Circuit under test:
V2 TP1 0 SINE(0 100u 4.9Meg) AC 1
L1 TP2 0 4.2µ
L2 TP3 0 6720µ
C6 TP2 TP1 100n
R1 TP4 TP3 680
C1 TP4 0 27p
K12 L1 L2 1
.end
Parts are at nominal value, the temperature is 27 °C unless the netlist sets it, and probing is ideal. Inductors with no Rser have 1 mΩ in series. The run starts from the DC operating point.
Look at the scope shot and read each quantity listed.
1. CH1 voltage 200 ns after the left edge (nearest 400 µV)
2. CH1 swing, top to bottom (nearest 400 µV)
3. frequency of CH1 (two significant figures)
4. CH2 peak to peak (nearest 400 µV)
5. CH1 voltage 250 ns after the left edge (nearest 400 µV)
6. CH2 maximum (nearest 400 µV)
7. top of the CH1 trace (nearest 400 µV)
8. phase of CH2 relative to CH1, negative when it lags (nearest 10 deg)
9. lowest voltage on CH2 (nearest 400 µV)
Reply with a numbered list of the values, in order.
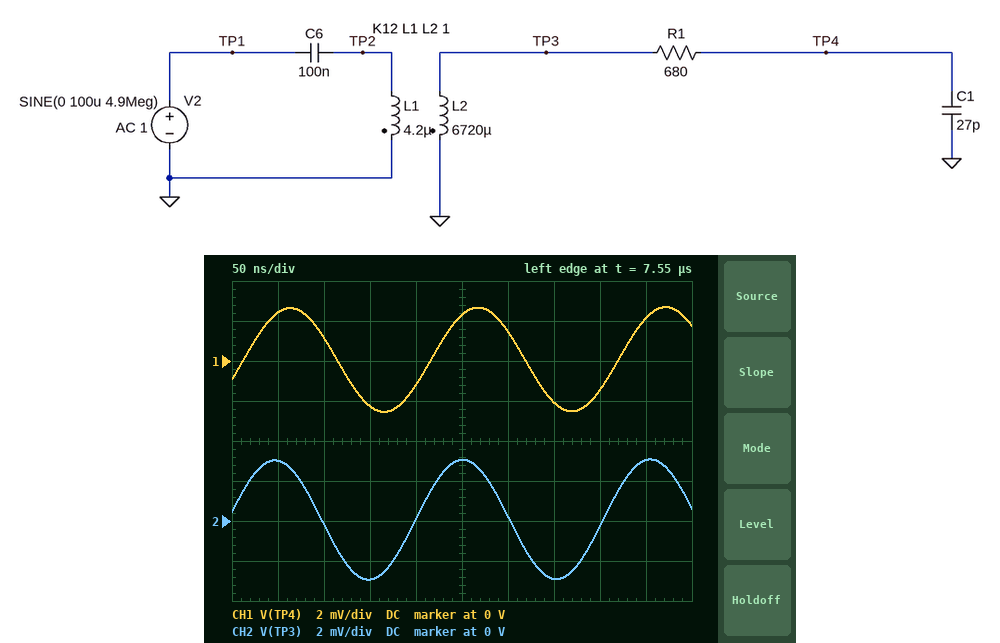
1. -1.2 mV
2. 5.2 mV
3. 4.9 MHz
4. 6.0 mV
5. 2.4 mV
6. 3.2 mV
7. 2.8 mV
8. 30 deg
9. -2.8 mV
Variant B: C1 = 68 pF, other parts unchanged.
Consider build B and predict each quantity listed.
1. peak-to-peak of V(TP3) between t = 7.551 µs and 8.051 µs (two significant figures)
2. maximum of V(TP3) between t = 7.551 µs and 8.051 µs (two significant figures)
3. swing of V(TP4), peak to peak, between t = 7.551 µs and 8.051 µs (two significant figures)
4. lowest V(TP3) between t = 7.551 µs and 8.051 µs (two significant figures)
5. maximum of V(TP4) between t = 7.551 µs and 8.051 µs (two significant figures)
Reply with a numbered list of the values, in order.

1. 5.5 mV
2. 2.7 mV
3. 3.2 mV
4. -2.8 mV
5. 1.5 mV
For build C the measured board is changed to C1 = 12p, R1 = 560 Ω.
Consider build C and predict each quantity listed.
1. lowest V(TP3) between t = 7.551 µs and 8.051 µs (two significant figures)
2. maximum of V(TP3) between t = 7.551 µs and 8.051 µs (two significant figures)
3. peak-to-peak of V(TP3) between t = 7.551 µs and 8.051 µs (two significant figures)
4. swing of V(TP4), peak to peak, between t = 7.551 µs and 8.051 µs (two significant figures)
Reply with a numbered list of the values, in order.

1. -3.2 mV
2. 3.5 mV
3. 6.8 mV
4. 6.6 mV
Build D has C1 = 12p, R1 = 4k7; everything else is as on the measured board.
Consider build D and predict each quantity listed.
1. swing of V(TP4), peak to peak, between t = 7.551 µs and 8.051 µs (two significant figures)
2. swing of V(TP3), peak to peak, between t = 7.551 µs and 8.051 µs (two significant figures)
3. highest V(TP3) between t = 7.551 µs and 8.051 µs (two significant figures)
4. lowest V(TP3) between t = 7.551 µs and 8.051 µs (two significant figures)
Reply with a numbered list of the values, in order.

1. 3.8 mV
2. 7.6 mV
3. 4.0 mV
4. -3.7 mV
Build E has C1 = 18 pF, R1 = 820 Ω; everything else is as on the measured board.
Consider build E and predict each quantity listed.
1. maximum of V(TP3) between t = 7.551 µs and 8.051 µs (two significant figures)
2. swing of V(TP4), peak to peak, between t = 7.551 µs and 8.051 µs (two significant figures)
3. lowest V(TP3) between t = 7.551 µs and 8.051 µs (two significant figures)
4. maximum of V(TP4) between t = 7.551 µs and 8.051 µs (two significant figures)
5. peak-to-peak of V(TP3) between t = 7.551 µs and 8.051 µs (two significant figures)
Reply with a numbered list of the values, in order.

1. 3.4 mV
2. 5.9 mV
3. -3.1 mV
4. 3.1 mV
5. 6.5 mV
